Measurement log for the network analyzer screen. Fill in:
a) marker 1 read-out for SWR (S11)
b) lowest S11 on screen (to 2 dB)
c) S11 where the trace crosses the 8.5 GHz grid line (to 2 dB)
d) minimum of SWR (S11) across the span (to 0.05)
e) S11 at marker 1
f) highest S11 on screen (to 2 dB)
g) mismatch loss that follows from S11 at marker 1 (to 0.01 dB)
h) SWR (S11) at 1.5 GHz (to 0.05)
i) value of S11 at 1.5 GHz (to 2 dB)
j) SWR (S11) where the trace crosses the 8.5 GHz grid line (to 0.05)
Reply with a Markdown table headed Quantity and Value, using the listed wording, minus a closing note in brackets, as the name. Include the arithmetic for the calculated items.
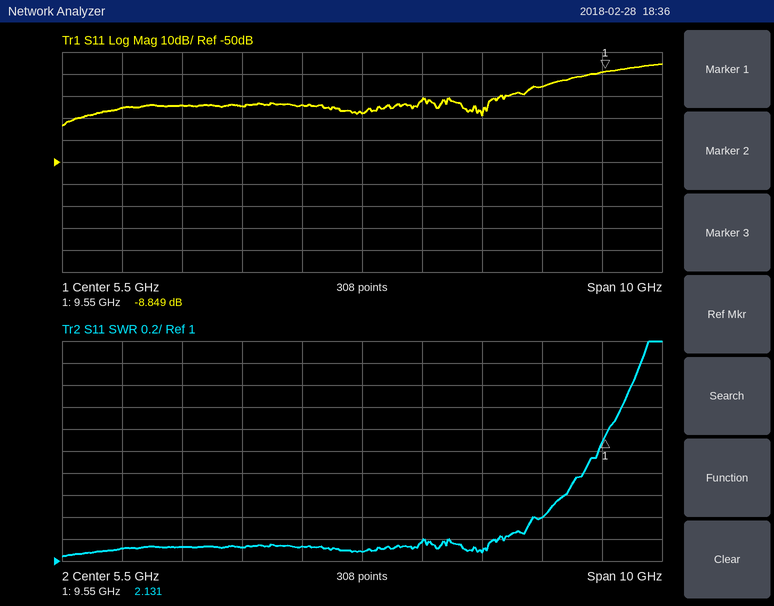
| Quantity | Value |
|---|---|
| marker 1 read-out for SWR | 2.131 |
| lowest S11 on screen | -34 dB |
| S11 where the trace crosses the 8.5 GHz grid line | -16 dB |
| minimum of SWR (S11) across the span | 1.05 |
| S11 at marker 1 | -8.849 dB |
| highest S11 on screen | -6 dB |
| mismatch loss that follows from S11 at marker 1 | −10 log10(1 − 10^(-8.849/10)) ≈ 0.61 dB |
| SWR (S11) at 1.5 GHz | 1.10 |
| value of S11 at 1.5 GHz | -26 dB |
| SWR (S11) where the trace crosses the 8.5 GHz grid line | 1.40 |
